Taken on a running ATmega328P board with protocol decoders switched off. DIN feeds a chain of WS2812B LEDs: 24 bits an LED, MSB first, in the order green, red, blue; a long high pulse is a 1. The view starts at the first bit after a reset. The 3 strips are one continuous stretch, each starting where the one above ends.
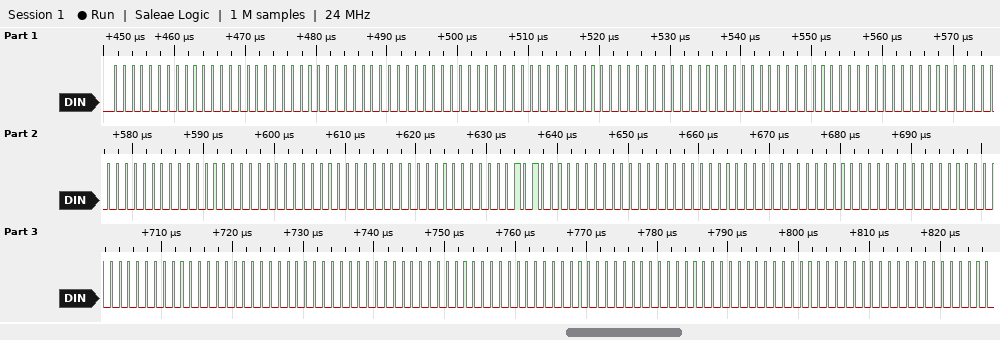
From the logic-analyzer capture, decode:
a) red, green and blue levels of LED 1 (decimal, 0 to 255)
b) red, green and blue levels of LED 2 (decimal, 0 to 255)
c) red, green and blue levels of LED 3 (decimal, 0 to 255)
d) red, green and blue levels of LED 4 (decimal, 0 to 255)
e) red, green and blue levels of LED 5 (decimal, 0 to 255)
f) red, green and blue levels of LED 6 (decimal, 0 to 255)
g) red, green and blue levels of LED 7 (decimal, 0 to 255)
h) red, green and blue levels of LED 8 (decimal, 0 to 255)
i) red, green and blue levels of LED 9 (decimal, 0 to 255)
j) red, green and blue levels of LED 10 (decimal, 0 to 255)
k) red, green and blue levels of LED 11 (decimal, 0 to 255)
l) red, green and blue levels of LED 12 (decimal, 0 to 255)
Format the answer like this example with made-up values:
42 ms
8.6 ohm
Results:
0, 0, 0
0, 0, 0
0, 0, 0
0, 0, 0
0, 0, 0
0, 0, 0
0, 40, 0
0, 0, 0
0, 0, 0
0, 0, 0
0, 0, 0
0, 0, 0
